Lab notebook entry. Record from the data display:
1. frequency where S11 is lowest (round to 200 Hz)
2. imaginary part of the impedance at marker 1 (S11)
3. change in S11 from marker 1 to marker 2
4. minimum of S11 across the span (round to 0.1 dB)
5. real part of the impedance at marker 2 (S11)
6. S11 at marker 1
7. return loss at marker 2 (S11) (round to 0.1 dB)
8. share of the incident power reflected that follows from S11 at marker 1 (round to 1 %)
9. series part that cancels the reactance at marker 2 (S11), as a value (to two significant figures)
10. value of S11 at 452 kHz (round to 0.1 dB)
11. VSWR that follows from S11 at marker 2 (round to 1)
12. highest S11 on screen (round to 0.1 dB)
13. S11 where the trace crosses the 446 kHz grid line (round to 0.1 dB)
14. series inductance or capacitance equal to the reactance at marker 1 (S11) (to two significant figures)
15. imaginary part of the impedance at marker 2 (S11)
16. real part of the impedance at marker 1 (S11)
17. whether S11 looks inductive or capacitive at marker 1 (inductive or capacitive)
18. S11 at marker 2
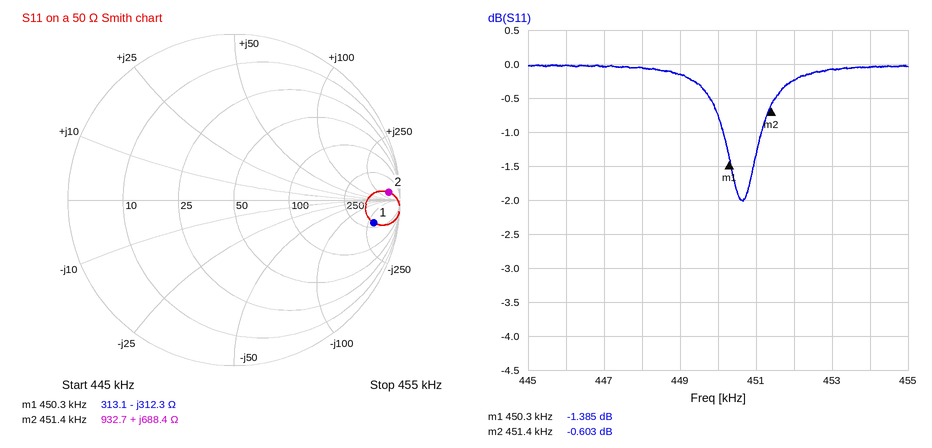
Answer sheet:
450.6 kHz
-312.3 Ω
0.782 dB
-2.0 dB
932.7 Ω
-1.385 dB
0.6 dB
73 %
510 pF
-0.2 dB
29
0.0 dB
0.0 dB
1.1 nF
+688.4 Ω
313.1 Ω
capacitive
-0.603 dB
